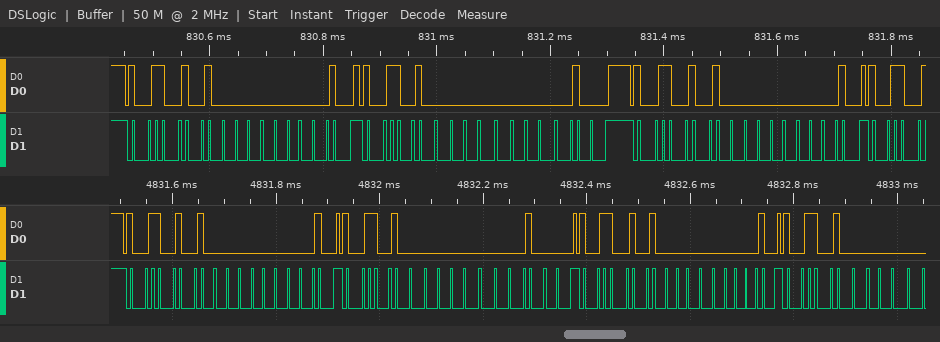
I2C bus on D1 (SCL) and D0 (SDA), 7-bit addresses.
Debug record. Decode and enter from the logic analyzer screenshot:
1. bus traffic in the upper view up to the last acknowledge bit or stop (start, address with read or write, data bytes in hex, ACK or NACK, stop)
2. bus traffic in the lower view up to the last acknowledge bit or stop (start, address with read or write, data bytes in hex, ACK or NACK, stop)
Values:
start, address 5A read ACK, 00 NACK, stop, start, address 5A write ACK, 01 ACK, stop, start, address 5A read ACK, 00 NACK, stop
start, address 5A read ACK, 00 NACK, stop, start, address 5A write ACK, 02 ACK, stop, start, address 5A read ACK, 00 NACK, stop, start, address 5A write ACK
